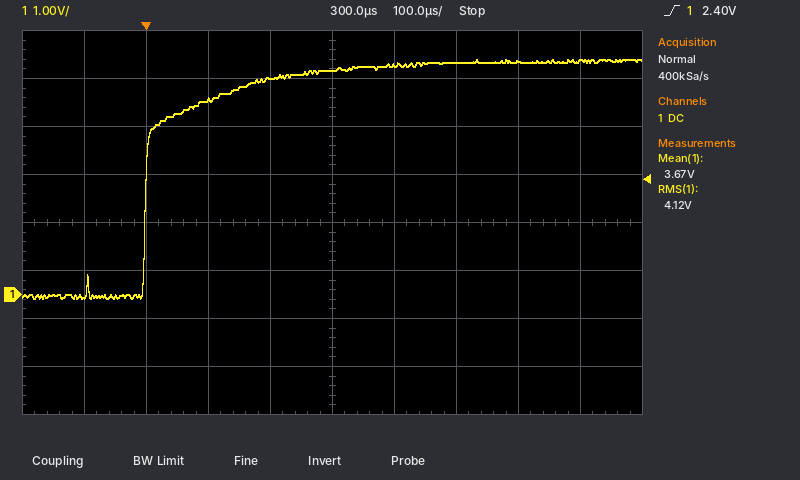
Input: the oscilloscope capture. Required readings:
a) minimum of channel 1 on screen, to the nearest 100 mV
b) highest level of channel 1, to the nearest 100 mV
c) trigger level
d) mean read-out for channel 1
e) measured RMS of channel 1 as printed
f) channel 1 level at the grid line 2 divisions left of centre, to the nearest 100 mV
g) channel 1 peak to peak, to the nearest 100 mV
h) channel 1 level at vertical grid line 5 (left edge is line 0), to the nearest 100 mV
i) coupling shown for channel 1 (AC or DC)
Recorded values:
-100 mV
4.9 V
2.40 V
3.67 V
4.12 V
4.1 V
5.0 V
4.7 V
DC
